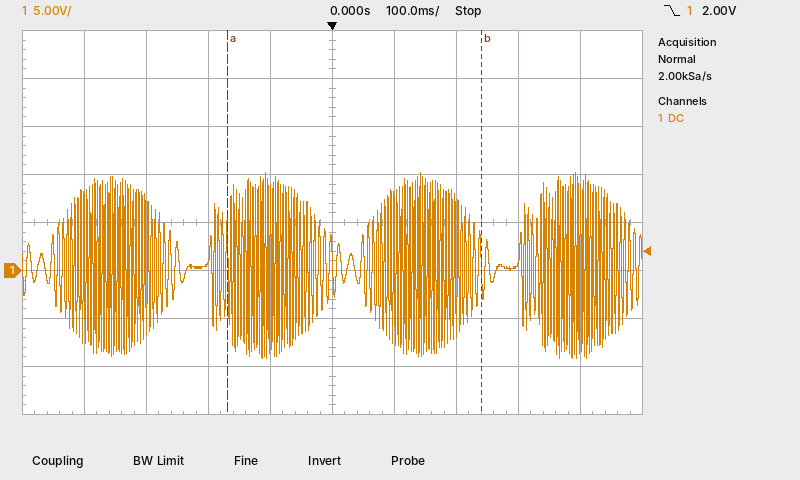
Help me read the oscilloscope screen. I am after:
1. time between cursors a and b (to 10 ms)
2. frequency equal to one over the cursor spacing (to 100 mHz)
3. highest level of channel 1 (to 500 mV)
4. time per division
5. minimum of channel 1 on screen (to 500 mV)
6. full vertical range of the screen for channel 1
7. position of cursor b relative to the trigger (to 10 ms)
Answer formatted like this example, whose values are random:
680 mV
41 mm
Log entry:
410 ms
2.4 Hz
10.0 V
100 ms
-9.0 V
40 V
+240 ms
